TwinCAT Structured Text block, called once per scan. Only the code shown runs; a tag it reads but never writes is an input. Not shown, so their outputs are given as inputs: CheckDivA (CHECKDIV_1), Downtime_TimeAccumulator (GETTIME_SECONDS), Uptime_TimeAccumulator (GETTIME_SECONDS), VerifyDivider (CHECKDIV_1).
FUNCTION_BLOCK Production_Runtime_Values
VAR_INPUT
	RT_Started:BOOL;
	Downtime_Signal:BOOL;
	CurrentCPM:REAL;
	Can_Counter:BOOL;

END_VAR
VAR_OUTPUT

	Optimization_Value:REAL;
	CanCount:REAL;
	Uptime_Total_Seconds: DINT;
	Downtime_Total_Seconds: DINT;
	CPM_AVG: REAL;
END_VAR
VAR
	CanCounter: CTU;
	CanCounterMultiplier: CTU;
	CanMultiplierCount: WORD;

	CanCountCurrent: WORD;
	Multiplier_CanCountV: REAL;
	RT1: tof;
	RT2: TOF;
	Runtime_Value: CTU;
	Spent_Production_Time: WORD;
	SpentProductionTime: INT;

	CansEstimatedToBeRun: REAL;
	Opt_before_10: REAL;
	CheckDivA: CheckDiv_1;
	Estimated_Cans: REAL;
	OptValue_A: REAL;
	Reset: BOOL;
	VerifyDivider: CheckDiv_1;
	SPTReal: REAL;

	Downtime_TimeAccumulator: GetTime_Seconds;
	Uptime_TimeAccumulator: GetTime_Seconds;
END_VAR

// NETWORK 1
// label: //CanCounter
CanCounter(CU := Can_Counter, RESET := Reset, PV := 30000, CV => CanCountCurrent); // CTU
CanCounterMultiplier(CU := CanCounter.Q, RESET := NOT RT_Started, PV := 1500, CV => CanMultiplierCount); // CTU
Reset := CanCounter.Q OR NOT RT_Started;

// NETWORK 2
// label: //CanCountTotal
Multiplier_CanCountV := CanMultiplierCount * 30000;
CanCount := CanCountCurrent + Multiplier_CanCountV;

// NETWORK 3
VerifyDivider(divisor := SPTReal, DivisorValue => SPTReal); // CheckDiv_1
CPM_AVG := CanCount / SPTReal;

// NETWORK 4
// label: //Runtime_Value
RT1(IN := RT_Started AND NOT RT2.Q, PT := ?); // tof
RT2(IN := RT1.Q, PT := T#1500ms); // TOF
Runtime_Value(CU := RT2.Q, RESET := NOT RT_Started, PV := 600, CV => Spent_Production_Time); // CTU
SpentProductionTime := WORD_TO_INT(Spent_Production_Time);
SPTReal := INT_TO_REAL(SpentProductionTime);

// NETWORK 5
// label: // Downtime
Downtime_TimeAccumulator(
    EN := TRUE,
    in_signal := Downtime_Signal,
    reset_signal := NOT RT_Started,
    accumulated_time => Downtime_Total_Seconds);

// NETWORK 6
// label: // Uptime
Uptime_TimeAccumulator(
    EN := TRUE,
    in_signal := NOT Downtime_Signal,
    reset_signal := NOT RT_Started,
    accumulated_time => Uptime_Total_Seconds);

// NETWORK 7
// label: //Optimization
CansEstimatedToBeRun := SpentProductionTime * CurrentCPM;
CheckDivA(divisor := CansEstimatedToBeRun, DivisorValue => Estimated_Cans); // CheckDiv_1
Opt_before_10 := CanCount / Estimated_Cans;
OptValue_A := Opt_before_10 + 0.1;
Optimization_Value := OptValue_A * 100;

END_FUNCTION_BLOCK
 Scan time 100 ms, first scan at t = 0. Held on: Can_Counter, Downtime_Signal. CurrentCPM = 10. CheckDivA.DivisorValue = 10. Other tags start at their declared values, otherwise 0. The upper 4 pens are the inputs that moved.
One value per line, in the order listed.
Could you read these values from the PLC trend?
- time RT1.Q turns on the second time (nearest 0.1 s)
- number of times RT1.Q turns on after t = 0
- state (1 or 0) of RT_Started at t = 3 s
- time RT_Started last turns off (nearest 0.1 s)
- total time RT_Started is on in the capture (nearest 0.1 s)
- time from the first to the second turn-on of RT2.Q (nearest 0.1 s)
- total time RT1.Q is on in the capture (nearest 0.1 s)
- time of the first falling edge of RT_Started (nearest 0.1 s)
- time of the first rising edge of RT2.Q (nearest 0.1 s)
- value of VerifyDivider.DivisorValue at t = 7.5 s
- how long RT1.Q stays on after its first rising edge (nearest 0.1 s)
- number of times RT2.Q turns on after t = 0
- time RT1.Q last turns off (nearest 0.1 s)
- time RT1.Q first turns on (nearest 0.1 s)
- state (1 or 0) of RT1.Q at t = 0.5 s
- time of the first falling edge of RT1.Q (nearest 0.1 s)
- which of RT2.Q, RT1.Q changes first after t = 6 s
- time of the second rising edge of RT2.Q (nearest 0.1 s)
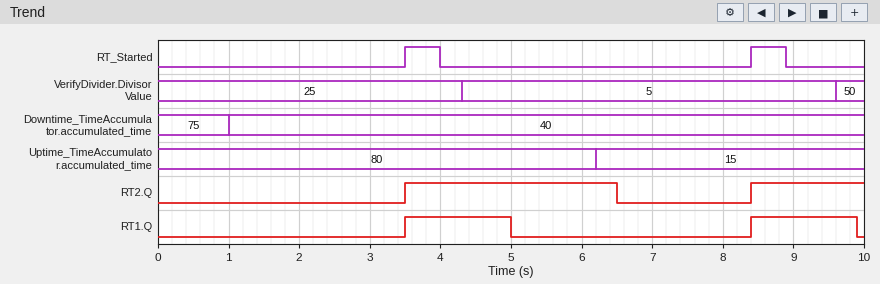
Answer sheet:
8.4 s
2
0
8.9 s
1.0 s
4.9 s
3.0 s
4.0 s
3.5 s
5
1.5 s
2
9.9 s
3.5 s
0
5.0 s
RT2.Q
8.4 s
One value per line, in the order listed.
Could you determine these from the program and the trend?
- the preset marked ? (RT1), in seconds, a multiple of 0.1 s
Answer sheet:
1.4 s
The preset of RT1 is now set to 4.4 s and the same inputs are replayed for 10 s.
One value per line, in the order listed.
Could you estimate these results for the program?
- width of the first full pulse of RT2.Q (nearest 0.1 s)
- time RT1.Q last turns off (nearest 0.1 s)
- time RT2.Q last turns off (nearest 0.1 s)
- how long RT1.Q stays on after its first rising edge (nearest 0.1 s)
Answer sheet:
6.0 s
8.0 s
9.5 s
4.5 s
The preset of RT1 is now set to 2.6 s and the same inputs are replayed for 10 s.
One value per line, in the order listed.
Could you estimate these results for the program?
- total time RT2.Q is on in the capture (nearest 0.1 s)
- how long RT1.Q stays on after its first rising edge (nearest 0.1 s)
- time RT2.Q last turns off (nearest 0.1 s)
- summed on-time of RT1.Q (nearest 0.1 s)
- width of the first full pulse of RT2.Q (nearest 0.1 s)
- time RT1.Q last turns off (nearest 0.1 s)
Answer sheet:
5.8 s
2.7 s
7.7 s
4.3 s
4.2 s
6.2 s
